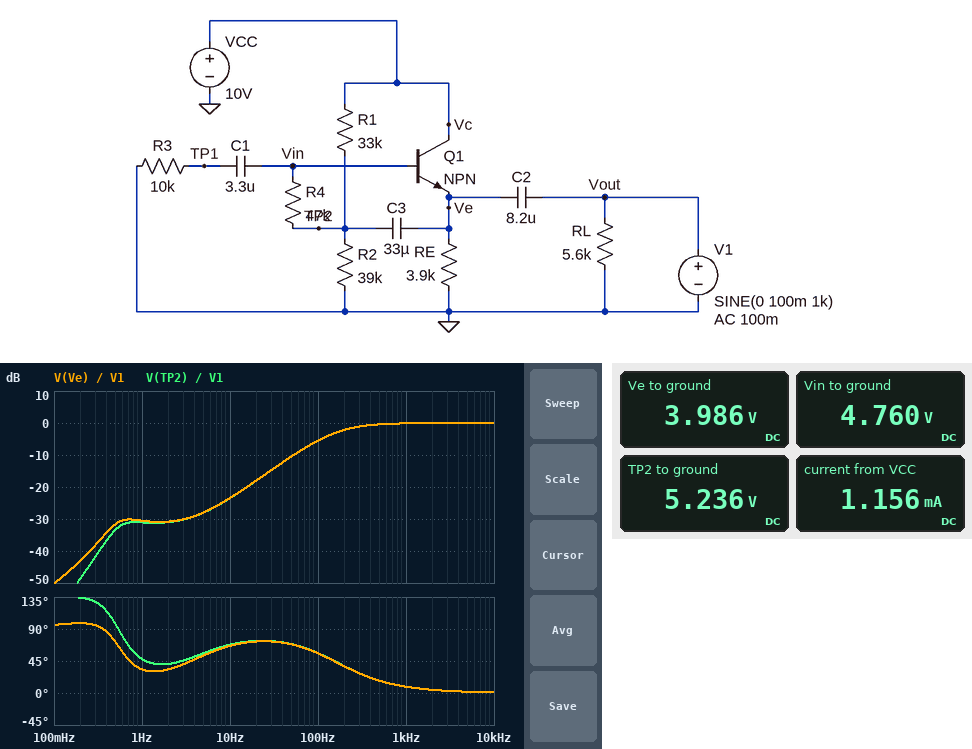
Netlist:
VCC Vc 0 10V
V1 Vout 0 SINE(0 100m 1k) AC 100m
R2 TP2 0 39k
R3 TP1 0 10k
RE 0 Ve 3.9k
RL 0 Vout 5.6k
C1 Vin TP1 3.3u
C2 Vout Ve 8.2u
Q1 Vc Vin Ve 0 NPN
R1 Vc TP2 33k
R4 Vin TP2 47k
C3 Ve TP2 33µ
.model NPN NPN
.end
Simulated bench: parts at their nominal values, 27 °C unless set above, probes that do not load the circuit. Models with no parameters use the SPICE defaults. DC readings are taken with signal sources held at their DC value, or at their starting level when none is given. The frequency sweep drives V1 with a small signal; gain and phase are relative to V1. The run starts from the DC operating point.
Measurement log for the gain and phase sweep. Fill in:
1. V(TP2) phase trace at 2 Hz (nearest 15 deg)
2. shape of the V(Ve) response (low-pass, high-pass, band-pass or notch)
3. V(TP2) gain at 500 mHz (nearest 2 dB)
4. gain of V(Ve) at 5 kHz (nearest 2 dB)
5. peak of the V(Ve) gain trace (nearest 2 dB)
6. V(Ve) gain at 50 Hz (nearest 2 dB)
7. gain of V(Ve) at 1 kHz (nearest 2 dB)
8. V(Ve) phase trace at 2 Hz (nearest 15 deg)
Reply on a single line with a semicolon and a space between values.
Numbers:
45 deg; high-pass; -34 dB; 0 dB; 0 dB; -10 dB; 0 dB; 30 deg
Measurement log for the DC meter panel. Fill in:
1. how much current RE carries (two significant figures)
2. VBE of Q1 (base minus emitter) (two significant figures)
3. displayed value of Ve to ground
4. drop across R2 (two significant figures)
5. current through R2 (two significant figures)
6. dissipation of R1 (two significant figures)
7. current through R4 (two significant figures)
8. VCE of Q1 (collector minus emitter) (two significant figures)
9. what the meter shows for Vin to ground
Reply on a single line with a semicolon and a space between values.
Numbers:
1.0 mA; 770 mV; 3.986 V; 5.2 V; 130 µA; 690 µW; 10 µA; 6.0 V; 4.760 V
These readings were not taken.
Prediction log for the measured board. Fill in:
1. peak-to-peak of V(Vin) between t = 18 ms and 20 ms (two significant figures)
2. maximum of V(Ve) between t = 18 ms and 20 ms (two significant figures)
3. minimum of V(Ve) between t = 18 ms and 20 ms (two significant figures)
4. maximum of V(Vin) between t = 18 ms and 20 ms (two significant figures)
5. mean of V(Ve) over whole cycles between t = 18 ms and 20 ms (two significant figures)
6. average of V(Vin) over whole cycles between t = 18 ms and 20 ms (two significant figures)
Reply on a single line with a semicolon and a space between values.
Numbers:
150 mV; 4.1 V; 3.9 V; 4.8 V; 4.0 V; 4.8 V
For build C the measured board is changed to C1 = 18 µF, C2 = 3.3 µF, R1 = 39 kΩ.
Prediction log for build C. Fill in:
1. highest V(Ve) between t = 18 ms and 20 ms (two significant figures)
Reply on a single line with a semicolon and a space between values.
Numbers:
3.7 V
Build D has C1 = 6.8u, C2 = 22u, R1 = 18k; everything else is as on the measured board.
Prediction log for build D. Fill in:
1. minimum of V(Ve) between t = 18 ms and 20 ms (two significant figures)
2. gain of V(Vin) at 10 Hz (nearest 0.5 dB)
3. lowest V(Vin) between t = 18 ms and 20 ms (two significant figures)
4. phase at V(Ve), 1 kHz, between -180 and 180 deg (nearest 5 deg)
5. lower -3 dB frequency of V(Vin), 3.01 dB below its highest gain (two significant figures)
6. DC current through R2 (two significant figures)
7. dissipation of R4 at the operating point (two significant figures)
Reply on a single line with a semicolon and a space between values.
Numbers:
5.2 V; -17.5 dB; 6.0 V; 5 deg; 63 Hz; 170 µA; 8.4 µW
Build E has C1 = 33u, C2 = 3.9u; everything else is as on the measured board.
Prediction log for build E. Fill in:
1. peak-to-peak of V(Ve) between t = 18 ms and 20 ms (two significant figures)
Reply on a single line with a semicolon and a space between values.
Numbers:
190 mV
